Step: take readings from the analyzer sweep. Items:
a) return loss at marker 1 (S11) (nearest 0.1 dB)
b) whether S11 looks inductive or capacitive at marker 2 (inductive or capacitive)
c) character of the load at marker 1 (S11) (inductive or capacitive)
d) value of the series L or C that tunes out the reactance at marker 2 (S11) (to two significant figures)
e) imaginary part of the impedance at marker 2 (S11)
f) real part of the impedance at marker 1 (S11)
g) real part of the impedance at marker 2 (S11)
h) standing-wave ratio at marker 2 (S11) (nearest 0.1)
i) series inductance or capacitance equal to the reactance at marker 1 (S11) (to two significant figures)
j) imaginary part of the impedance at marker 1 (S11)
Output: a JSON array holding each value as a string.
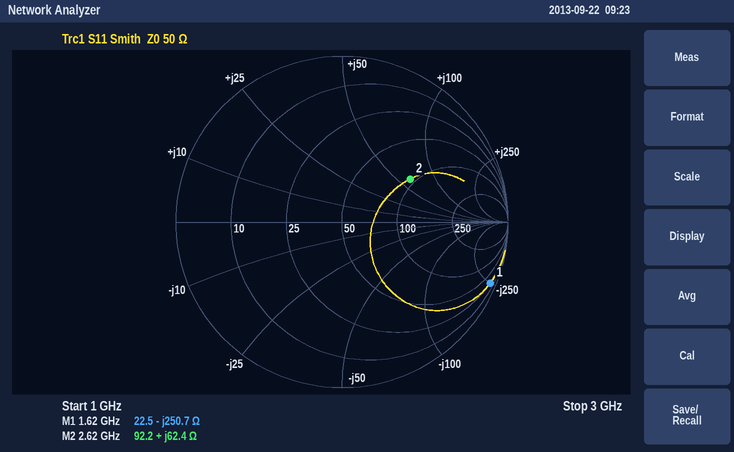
["0.3 dB", "inductive", "capacitive", "970 fF", "+62.4 Ω", "22.5 Ω", "92.2 Ω", "2.9", "390 fF", "-250.7 Ω"]
